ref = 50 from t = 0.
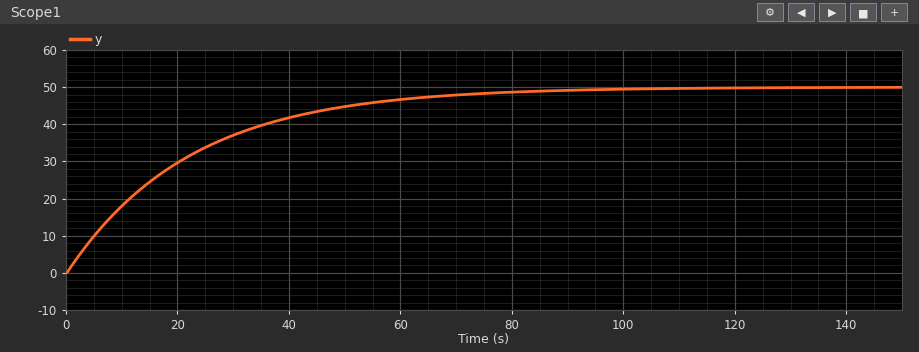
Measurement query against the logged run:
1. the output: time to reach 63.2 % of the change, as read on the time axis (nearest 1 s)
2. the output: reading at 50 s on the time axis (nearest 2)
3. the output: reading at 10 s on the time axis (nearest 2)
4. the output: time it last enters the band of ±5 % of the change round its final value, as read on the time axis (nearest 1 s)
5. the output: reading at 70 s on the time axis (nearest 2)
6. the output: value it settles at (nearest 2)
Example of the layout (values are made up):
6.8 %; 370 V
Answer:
22 s; 44; 18; 66 s; 48; 50
